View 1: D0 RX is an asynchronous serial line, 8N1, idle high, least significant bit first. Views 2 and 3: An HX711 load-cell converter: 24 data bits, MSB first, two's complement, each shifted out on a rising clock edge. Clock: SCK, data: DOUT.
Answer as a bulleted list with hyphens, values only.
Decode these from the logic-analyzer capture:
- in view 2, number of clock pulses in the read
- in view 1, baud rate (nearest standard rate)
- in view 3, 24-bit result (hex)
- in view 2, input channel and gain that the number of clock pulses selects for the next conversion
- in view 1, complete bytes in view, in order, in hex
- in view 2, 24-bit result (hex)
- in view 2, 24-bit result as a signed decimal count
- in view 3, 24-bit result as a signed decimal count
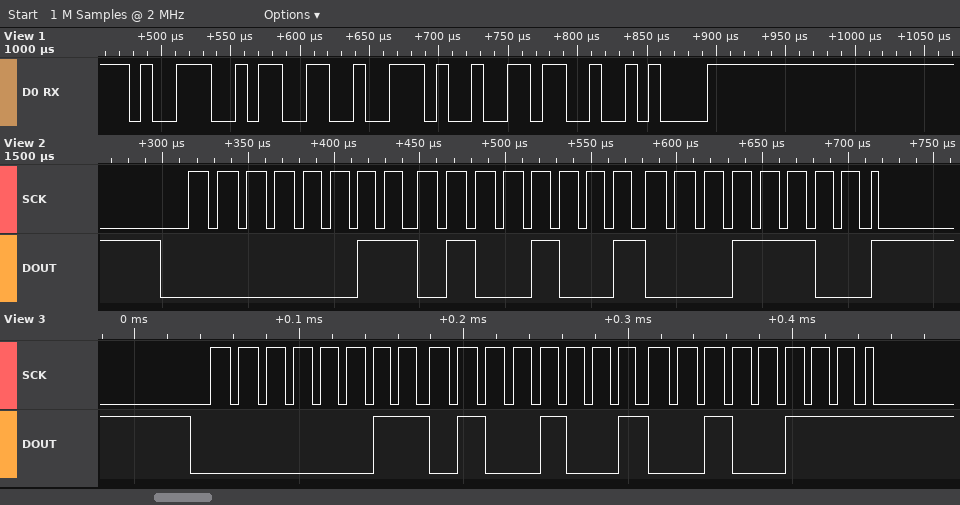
- 25
- 115200 baud
- 0x034927
- channel A, gain 128
- 39 33 2E 36 0A
- 0x03491C
- 215324
- 215335
